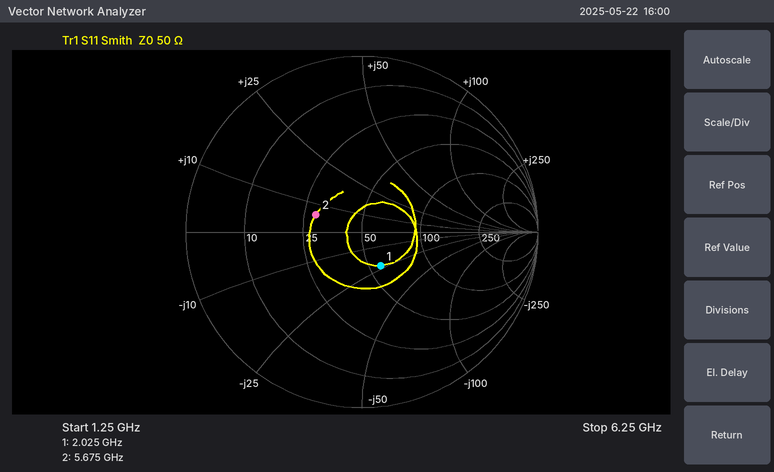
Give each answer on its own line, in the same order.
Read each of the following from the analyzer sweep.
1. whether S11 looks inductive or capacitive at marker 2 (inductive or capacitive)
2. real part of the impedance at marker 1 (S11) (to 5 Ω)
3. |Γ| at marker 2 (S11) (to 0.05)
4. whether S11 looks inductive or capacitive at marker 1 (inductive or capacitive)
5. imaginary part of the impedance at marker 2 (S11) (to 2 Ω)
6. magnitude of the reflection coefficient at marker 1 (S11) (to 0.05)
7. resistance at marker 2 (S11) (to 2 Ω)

inductive
55 Ω
0.30
capacitive
+6 Ω
0.20
28 Ω
